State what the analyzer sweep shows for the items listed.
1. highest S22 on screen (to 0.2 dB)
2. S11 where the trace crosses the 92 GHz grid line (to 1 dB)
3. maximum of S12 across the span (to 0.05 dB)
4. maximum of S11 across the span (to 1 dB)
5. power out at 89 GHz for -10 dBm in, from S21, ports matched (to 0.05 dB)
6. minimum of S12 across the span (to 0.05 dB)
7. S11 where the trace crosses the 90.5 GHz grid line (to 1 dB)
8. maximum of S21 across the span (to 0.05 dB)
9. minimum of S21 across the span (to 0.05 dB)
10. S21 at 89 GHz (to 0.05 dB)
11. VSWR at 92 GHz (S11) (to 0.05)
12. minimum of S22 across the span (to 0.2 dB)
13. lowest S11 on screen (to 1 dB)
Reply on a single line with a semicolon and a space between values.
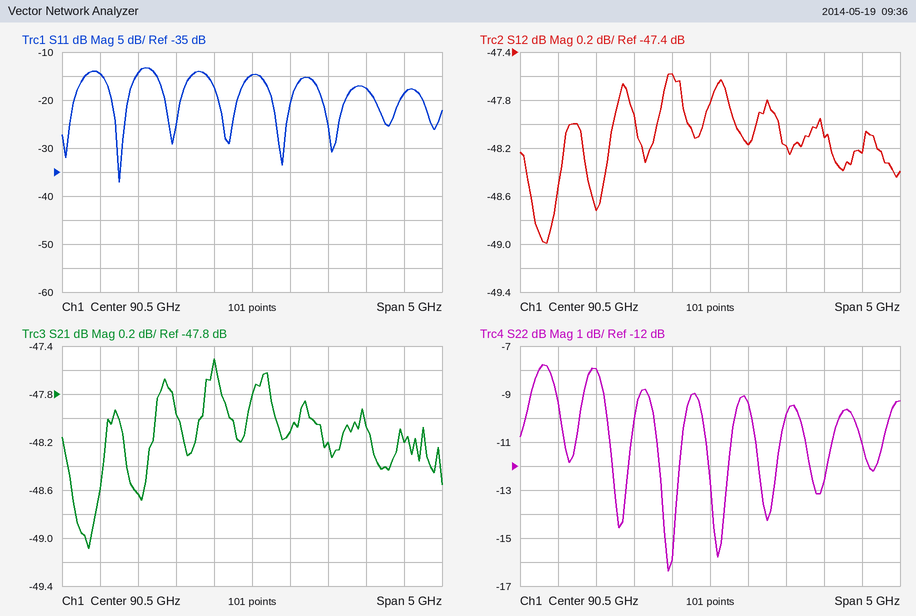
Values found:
-7.8 dB; -18 dB; -47.60 dB; -13 dB; -58.65 dBm; -49.00 dB; -15 dB; -47.50 dB; -49.10 dB; -48.65 dB; 1.30; -16.4 dB; -37 dB
